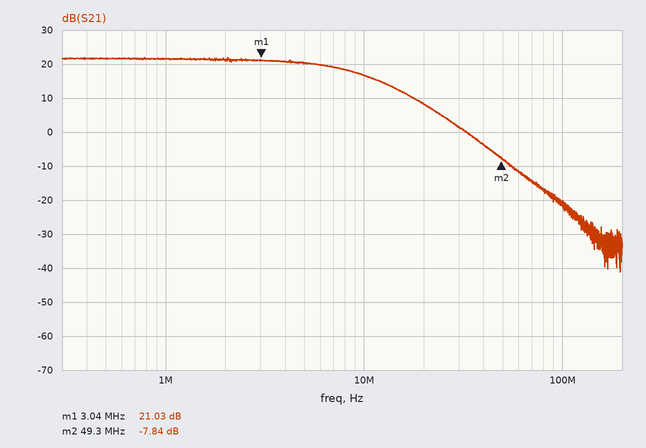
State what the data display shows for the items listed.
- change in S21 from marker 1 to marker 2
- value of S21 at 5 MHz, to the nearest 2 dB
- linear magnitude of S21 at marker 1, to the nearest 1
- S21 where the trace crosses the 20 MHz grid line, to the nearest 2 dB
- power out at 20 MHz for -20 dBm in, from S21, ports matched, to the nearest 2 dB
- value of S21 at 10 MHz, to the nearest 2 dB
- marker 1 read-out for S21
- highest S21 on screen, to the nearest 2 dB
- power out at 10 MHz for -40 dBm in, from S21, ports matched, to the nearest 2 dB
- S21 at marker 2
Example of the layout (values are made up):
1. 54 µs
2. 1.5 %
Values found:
1. -28.87 dB
2. 20 dB
3. 11
4. 8 dB
5. -12 dBm
6. 16 dB
7. 21.03 dB
8. 22 dB
9. -24 dBm
10. -7.84 dB
